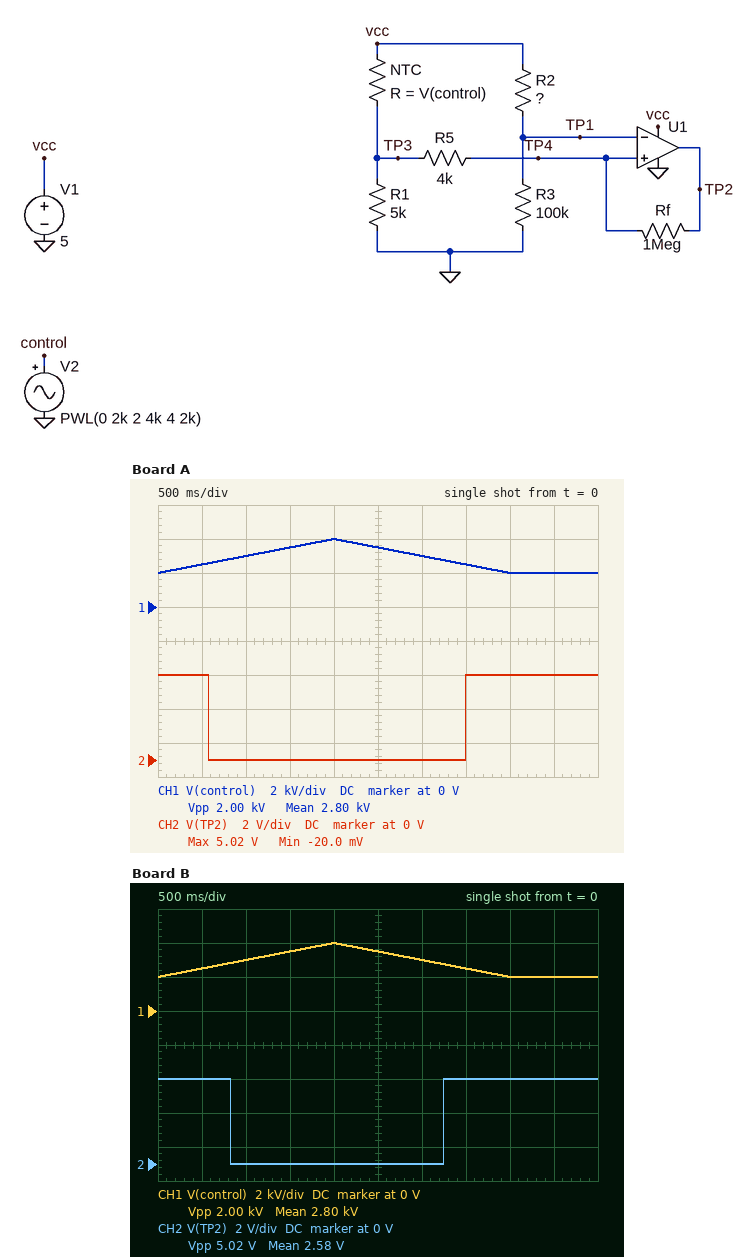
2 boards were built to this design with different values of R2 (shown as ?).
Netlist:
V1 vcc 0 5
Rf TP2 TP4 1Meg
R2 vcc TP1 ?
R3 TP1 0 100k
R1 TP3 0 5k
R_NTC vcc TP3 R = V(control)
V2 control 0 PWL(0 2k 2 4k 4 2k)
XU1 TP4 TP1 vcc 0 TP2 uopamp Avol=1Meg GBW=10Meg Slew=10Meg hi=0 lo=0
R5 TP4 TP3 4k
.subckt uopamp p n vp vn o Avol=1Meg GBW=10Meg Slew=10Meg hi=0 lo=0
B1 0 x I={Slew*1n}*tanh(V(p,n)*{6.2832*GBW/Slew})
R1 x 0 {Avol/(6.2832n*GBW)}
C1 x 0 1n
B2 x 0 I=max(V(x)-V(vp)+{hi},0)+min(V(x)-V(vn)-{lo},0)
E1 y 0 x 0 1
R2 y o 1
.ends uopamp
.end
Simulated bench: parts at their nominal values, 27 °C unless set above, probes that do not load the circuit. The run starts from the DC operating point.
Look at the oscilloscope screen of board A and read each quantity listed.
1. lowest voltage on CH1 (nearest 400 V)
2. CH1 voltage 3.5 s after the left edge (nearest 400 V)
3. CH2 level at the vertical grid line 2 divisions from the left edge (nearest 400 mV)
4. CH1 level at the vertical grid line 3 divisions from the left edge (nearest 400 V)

2.0 kV
2.4 kV
0 V
3.6 kV
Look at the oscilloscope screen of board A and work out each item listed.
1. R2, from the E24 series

51 kΩ
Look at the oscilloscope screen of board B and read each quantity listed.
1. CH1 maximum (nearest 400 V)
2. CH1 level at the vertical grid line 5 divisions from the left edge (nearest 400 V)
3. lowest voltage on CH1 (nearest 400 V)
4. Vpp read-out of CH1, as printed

4.0 kV
3.6 kV
2.0 kV
2.00 kV
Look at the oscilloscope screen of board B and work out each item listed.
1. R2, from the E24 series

56 kΩ
